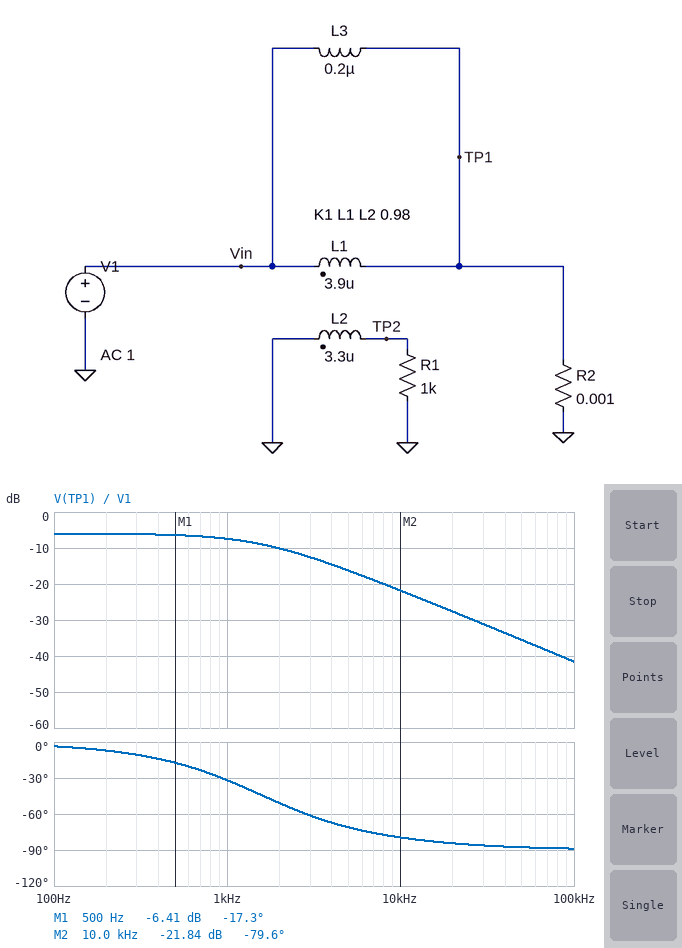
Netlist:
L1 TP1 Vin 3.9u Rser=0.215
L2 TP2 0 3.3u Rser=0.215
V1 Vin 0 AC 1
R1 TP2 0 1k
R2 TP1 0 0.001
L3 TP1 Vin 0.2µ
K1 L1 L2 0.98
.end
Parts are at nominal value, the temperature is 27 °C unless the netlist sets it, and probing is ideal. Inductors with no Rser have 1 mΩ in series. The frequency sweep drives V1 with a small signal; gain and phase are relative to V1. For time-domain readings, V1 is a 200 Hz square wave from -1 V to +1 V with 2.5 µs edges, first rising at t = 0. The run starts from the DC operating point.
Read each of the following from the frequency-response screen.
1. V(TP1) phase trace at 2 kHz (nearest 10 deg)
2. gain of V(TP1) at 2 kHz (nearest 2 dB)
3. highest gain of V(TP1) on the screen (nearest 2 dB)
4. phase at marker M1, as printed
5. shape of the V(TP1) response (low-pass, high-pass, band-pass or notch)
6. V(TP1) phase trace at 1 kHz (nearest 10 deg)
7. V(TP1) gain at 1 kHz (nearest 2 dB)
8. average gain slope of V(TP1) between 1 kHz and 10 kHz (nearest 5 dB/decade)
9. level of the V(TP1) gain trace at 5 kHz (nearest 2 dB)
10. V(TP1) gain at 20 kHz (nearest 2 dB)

-50 deg
-10 dB
-6 dB
-17.3 deg
low-pass
-30 deg
-8 dB
-15 dB/decade
-16 dB
-28 dB
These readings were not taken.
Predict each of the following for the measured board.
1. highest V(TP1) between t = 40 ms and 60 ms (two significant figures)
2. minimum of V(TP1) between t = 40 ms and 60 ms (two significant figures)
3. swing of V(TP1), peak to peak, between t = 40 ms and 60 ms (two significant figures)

500 mV
-500 mV
1.0 V
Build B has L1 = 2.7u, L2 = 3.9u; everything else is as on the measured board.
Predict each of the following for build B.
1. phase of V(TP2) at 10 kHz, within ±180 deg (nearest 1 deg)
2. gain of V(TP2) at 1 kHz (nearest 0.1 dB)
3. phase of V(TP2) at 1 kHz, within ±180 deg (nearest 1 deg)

-124 deg
-24.0 dB
-75 deg
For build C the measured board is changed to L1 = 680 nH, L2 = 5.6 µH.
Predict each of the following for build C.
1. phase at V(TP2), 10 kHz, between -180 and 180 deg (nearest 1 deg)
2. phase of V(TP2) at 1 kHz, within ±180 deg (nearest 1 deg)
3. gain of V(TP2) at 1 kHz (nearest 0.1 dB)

-97 deg
-72 deg
-28.4 dB
